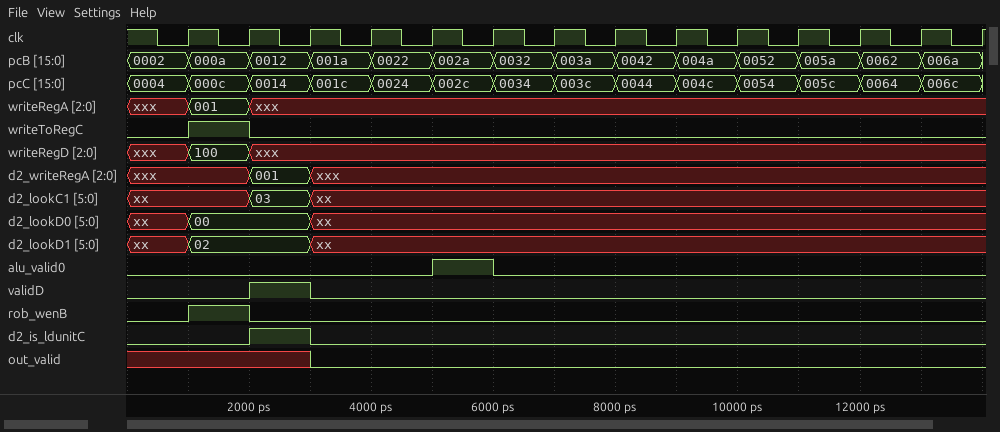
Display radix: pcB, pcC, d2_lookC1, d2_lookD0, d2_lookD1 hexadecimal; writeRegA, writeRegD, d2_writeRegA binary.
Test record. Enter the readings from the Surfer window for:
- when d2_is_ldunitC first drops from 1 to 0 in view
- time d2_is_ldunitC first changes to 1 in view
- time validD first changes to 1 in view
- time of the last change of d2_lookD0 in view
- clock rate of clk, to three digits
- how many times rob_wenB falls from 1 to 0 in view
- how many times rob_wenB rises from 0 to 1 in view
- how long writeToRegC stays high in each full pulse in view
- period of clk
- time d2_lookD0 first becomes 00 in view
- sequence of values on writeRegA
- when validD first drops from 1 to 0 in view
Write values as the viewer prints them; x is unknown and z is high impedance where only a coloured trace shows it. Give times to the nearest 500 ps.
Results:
3000 ps
2000 ps
2000 ps
3000 ps
1.00 GHz
1
1
1000 ps
1000 ps
1000 ps
xxx, 001, xxx
3000 ps
